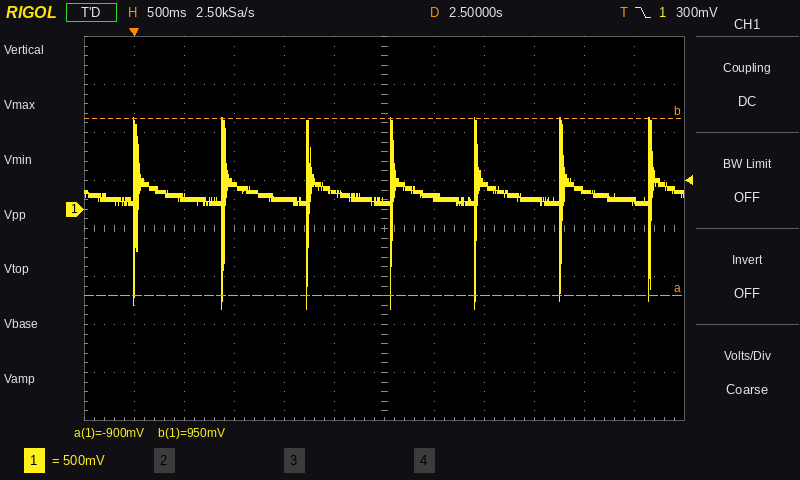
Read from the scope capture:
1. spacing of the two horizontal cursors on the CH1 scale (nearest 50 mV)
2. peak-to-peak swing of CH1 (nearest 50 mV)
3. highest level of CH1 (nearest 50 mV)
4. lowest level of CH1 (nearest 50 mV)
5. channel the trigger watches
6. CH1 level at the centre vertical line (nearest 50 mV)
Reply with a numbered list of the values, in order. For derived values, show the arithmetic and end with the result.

1. 1.85 V
2. 950 mV − (-1.05 V) = 2.00 V
3. 950 mV
4. -1.05 V
5. CH1
6. 100 mV
